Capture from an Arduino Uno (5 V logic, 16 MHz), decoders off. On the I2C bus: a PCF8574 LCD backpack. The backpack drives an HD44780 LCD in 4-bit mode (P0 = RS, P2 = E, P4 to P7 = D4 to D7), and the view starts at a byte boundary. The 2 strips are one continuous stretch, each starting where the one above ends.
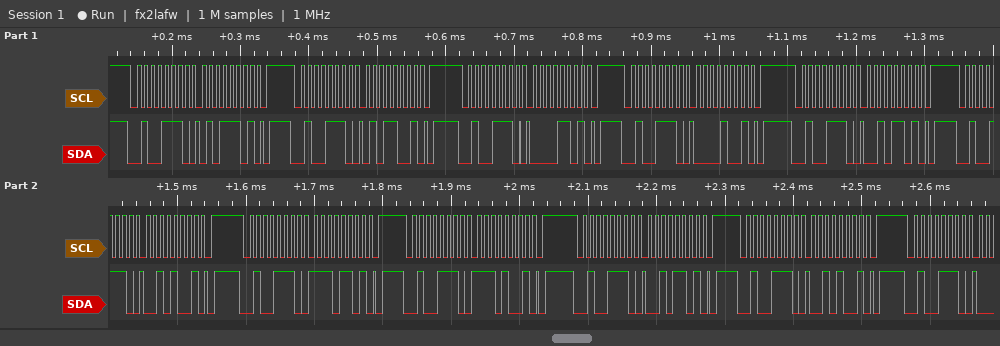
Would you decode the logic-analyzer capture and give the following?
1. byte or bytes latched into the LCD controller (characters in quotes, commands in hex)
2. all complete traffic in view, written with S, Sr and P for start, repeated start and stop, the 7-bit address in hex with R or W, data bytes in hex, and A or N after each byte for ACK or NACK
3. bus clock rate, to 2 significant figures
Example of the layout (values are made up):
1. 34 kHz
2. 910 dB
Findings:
1. 'P' '.'
2. S 27W A 5D A P S 27W A 59 A P S 27W A 0D A P S 27W A 09 A P S 27W A 2D A P S 27W A 29 A P S 27W A ED A P S 27W A E9 A P S 27W A 2D A P S 27W A 29 A P S 27W A
3. 100 kHz
